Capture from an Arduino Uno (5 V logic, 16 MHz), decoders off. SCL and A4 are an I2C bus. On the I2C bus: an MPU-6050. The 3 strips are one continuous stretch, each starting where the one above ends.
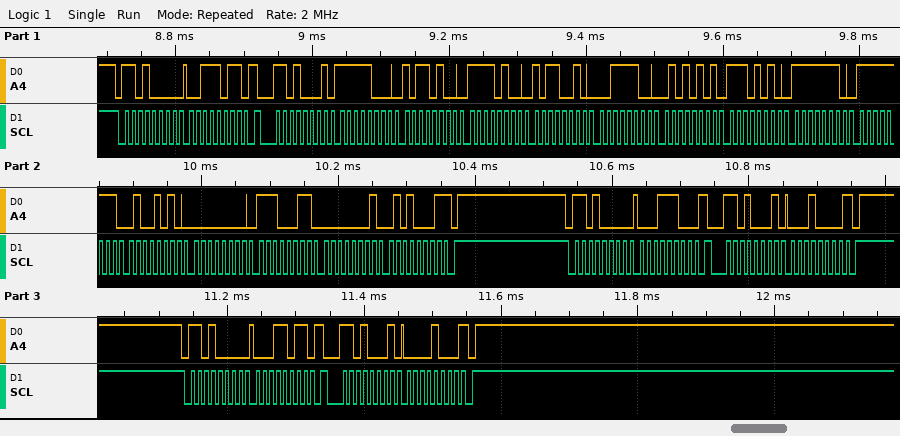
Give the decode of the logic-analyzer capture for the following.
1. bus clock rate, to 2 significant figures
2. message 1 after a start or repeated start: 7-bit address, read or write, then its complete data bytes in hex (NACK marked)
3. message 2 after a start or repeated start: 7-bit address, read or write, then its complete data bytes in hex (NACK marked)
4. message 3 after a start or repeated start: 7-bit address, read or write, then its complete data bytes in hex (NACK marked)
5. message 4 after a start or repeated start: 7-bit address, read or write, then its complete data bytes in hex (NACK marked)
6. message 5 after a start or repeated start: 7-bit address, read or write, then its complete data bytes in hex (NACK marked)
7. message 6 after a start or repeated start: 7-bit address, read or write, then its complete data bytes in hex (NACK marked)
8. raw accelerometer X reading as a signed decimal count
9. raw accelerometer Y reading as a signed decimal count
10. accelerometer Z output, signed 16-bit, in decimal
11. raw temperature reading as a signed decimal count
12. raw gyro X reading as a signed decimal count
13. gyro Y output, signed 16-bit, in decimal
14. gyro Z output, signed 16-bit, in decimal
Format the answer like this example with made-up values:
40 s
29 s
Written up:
100 kHz
0x68 write: 3B
0x68 read: F8 B4 F4 B2 3C 55 EA FE FF 4A 00 E3 01 51 NACK
0x68 write: 1C
0x68 read: 10 NACK
0x68 write: 1B
0x68 read: 08 NACK
-1868
-2894
15445
-5378
-182
227
337
